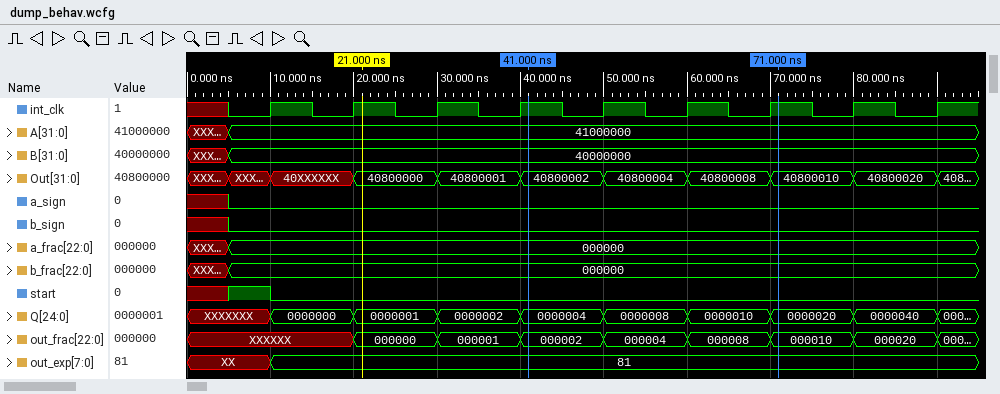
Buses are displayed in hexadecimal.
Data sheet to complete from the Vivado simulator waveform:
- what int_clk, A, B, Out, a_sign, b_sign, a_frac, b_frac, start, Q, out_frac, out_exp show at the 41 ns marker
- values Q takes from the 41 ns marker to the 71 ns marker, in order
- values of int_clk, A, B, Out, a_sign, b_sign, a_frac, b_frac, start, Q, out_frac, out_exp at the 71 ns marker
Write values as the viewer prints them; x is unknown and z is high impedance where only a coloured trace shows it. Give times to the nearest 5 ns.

int_clk=1, A=41000000, B=40000000, Out=40800002, a_sign=0, b_sign=0, a_frac=000000, b_frac=000000, start=0, Q=0000004, out_frac=000002, out_exp=81
0000004, 0000008, 0000010, 0000020
int_clk=1, A=41000000, B=40000000, Out=40800010, a_sign=0, b_sign=0, a_frac=000000, b_frac=000000, start=0, Q=0000020, out_frac=000010, out_exp=81
